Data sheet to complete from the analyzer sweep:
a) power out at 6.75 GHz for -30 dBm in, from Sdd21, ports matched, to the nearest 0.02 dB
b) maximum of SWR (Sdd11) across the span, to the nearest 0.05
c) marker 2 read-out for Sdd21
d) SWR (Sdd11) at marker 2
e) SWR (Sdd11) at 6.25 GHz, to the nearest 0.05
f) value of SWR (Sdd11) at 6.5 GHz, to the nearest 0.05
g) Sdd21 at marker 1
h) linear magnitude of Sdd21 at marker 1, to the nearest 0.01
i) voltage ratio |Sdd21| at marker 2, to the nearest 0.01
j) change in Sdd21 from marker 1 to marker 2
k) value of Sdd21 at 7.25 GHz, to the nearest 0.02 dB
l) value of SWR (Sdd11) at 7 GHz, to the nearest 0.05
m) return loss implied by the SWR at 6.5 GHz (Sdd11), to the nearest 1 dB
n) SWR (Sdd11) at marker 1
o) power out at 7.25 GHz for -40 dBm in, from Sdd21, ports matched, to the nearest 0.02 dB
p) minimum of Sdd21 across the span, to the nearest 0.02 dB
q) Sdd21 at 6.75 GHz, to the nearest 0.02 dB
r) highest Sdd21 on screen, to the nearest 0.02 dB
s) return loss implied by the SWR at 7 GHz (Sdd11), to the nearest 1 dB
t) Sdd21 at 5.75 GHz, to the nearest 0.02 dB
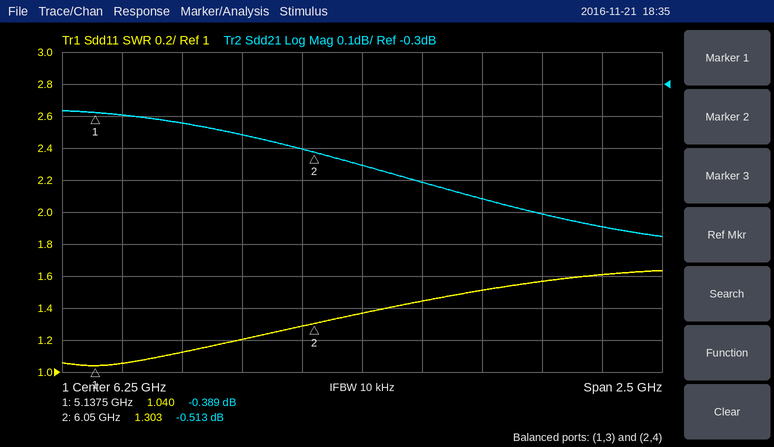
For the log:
-30.66 dBm
1.65
-0.513 dB
1.303
1.35
1.45
-0.389 dB
0.96
0.94
-0.124 dB
-0.74 dB
1.55
15 dB
1.040
-40.74 dBm
-0.78 dB
-0.66 dB
-0.38 dB
13 dB
-0.46 dB
